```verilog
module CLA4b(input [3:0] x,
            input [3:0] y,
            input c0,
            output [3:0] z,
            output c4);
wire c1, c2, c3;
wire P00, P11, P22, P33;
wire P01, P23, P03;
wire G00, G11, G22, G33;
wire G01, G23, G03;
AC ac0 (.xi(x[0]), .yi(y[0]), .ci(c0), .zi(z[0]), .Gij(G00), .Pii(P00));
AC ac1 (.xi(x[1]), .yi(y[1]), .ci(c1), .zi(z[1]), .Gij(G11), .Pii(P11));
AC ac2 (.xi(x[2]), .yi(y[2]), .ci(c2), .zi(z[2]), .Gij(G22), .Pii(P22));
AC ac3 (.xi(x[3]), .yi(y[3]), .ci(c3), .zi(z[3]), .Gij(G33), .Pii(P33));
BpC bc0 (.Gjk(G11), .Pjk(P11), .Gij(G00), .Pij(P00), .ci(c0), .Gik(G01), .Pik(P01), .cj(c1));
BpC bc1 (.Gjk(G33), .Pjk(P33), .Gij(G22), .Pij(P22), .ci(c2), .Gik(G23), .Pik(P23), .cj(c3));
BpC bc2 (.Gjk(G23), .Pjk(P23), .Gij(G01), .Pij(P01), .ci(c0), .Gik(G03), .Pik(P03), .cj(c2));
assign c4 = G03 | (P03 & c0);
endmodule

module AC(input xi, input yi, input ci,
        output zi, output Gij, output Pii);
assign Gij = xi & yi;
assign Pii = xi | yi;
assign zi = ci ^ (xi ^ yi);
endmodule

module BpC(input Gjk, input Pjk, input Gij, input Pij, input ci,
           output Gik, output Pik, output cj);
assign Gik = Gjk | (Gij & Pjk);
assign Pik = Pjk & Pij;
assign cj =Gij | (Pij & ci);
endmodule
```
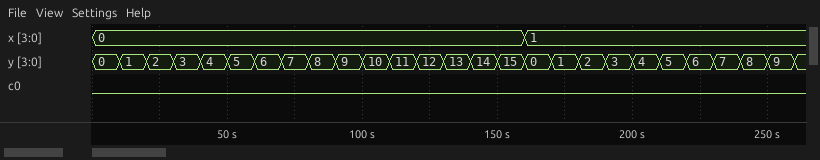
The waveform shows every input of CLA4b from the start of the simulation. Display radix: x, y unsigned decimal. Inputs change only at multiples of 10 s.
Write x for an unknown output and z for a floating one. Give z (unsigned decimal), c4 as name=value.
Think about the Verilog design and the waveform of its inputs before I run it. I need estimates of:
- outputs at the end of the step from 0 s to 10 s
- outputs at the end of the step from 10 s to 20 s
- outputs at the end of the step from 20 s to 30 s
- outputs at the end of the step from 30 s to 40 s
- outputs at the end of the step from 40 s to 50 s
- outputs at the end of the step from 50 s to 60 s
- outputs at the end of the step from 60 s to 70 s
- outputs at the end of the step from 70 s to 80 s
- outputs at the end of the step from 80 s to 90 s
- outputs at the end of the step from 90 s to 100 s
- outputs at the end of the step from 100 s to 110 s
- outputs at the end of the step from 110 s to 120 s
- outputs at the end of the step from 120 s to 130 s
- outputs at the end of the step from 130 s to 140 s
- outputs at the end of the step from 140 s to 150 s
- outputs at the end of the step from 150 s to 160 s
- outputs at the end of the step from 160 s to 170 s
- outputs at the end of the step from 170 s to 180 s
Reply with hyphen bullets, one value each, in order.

- z=0, c4=0
- z=1, c4=0
- z=2, c4=0
- z=3, c4=0
- z=4, c4=0
- z=5, c4=0
- z=6, c4=0
- z=7, c4=0
- z=8, c4=0
- z=9, c4=0
- z=10, c4=0
- z=11, c4=0
- z=12, c4=0
- z=13, c4=0
- z=14, c4=0
- z=15, c4=0
- z=1, c4=0
- z=2, c4=0
